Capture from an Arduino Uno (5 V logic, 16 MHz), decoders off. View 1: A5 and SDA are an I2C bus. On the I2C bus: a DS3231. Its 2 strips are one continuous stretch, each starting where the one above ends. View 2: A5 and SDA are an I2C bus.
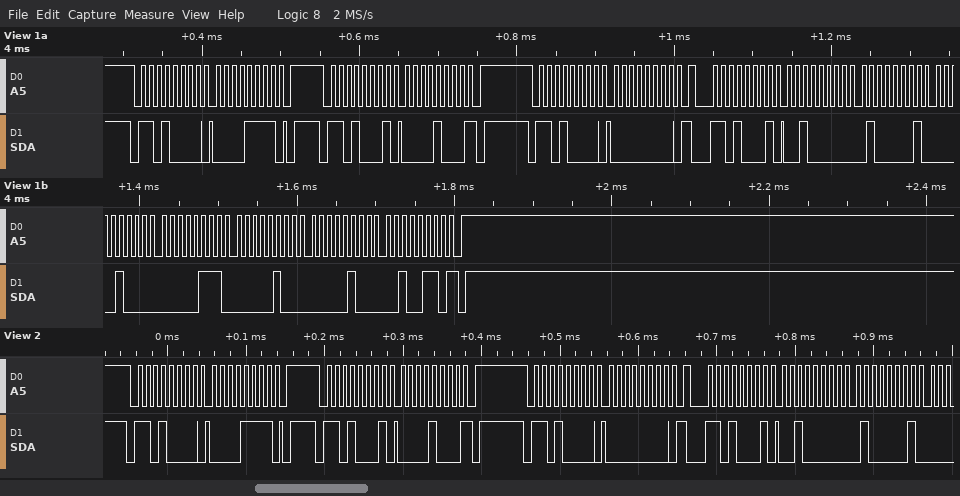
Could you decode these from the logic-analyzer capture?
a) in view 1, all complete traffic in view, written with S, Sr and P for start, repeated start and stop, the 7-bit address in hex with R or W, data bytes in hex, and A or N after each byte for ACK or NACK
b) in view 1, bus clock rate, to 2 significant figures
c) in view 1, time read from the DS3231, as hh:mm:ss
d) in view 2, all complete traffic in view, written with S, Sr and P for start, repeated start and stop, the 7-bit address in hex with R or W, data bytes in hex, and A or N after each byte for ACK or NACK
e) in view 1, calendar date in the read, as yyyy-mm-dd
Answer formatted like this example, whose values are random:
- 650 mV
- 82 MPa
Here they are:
- S 68W A 0F A P S 68R A 08 N P S 68W A 00 A Sr 68R A 20 A 41 A 08 A 07 A 04 A 04 A 26 N P
- 100 kHz
- 08:41:20
- S 68W A 0F A P S 68R A 08 N P S 68W A 00 A Sr 68R A 20 A 41 A
- 2026-04-04
